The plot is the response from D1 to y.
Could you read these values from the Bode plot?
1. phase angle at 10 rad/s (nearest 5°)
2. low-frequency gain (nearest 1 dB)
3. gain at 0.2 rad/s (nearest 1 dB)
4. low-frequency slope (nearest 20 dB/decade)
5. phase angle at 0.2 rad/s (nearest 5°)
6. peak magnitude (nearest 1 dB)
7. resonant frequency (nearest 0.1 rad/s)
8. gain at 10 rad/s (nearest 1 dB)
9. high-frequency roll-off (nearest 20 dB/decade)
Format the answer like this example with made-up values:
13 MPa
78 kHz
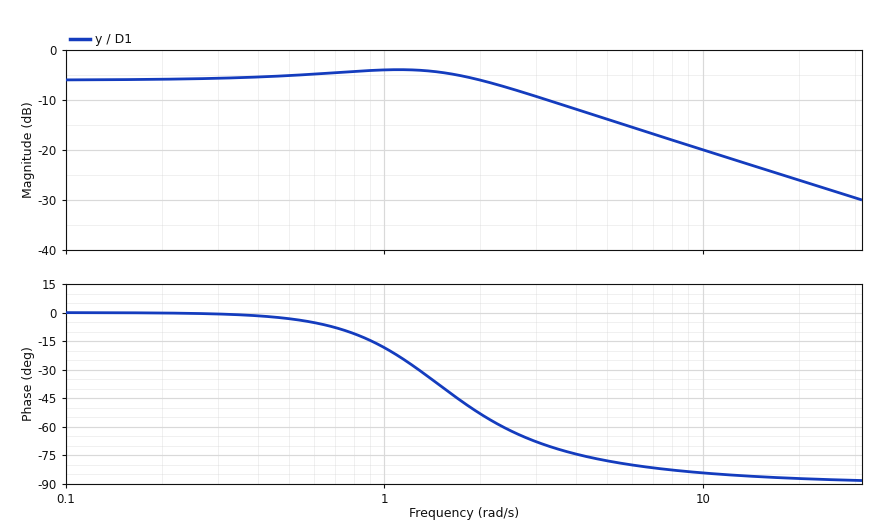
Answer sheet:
-85°
-6 dB
-6 dB
0 dB/decade
0°
-4 dB
1.1 rad/s
-20 dB
-20 dB/decade
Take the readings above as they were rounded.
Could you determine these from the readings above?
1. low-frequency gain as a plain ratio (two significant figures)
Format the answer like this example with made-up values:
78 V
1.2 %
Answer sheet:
0.50
